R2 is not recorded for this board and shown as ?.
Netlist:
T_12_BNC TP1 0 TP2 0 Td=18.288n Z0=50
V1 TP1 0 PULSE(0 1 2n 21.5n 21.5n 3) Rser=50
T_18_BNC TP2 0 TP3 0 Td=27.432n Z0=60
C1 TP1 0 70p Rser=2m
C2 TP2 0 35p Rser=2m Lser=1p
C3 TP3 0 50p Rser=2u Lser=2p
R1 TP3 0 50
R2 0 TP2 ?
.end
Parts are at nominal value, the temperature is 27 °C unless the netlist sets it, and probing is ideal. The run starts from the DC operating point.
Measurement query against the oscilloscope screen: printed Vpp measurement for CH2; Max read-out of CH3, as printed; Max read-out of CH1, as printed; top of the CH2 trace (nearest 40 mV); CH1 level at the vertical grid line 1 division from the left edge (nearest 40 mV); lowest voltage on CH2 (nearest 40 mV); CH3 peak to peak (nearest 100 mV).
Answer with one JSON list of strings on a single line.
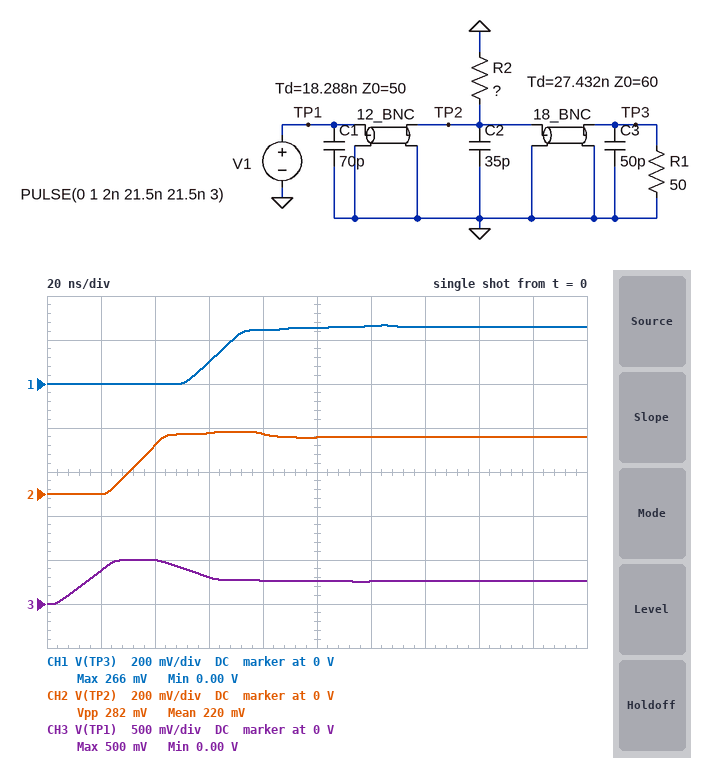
["282 mV", "500 mV", "266 mV", "280 mV", "0 V", "0 V", "500 mV"]
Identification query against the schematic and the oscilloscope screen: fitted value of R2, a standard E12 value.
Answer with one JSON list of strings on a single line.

["27 Ω"]
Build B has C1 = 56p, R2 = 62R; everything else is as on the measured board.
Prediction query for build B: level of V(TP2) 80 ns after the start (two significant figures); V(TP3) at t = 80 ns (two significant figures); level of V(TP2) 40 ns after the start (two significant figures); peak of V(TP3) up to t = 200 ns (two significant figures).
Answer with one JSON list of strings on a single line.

["370 mV", "340 mV", "310 mV", "360 mV"]
